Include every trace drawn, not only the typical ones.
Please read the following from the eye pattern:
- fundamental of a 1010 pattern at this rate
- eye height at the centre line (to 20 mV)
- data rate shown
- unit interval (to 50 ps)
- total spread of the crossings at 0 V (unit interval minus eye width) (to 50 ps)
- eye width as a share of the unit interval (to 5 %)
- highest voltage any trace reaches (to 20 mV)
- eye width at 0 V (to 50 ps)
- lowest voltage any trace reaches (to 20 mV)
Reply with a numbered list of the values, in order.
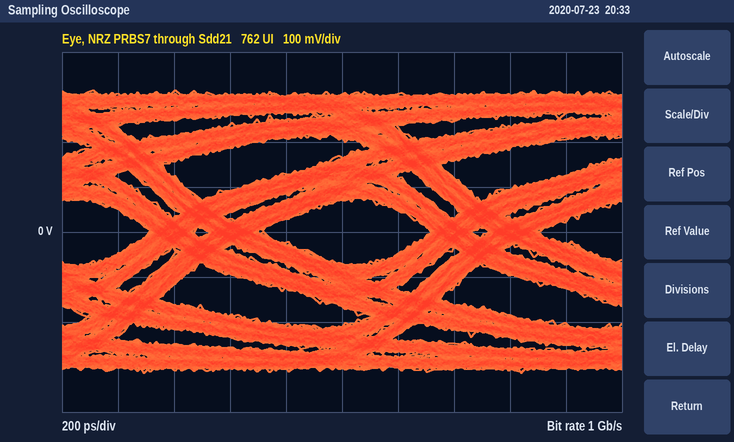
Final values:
1. 500 MHz
2. 140 mV
3. 1 Gb/s
4. 1.00 ns
5. 400 ps
6. 60 %
7. 320 mV
8. 600 ps
9. -320 mV
